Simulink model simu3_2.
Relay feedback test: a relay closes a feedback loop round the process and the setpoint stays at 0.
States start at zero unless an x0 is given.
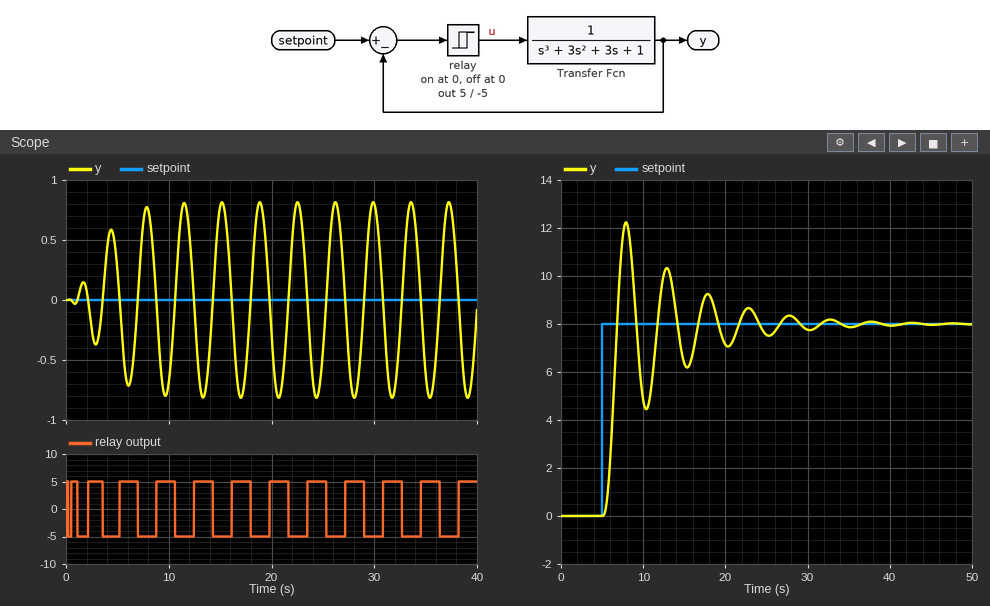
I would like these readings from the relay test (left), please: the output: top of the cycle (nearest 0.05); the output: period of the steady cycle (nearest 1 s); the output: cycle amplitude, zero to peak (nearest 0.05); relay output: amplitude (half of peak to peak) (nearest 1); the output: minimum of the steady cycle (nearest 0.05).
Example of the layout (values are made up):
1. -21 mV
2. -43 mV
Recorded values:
1. 0.80
2. 4 s
3. 0.80
4. 5
5. -0.80
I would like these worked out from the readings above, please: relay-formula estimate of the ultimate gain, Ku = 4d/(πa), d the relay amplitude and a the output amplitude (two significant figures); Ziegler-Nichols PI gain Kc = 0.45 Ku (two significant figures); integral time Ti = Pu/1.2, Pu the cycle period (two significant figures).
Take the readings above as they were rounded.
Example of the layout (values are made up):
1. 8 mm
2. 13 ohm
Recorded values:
1. 8.0
2. 3.6
3. 3.3 s
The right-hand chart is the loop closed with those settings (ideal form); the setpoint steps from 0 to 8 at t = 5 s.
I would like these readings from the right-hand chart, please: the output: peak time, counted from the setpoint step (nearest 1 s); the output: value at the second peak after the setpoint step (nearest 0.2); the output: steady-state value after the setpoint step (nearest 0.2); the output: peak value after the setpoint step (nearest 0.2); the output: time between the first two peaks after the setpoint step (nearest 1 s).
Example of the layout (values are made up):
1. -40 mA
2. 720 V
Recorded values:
1. 3 s
2. 10.4
3. 8.0
4. 12.2
5. 5 s
